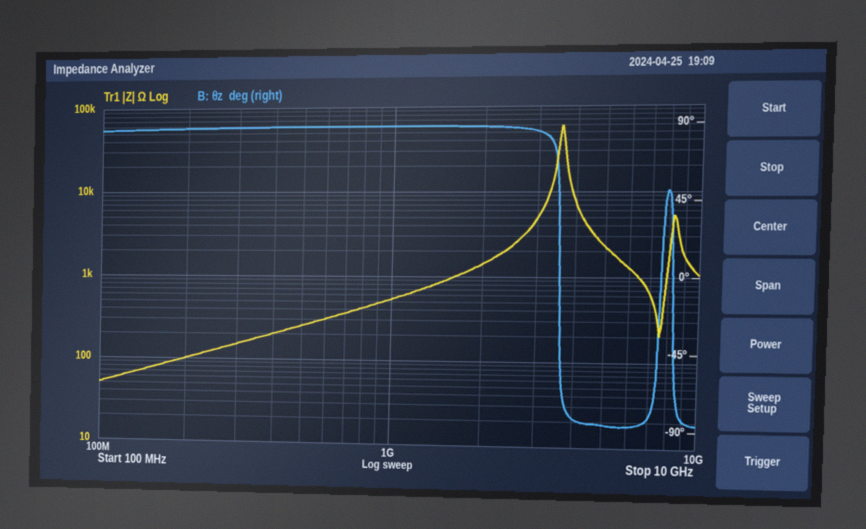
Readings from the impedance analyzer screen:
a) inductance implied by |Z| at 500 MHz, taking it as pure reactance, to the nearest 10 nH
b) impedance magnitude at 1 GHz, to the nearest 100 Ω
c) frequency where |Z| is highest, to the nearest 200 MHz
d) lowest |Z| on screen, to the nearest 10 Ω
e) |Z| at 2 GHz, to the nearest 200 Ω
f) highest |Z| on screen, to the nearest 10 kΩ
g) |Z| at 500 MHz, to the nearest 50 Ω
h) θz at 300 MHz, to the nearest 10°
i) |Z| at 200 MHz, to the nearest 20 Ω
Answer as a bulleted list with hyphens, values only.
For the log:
- 80 nH
- 500 Ω
- 3.6 GHz
- 50 Ω
- 1.4 kΩ
- 60 kΩ
- 250 Ω
- 90°
- 100 Ω
